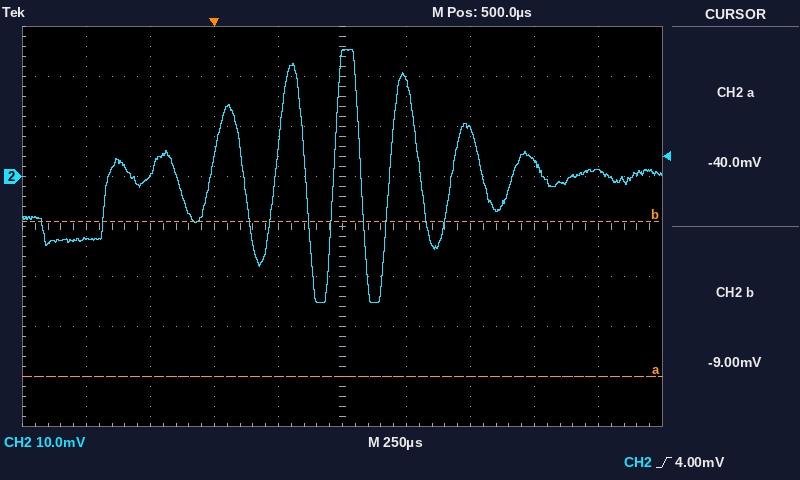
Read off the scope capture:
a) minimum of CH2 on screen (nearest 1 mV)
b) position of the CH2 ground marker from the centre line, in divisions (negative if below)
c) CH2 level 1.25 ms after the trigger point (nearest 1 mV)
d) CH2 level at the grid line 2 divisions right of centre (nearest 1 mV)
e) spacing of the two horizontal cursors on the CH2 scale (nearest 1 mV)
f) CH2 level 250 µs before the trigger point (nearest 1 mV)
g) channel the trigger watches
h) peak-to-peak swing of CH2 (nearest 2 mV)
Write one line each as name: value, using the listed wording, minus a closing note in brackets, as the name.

minimum of CH2 on screen: -25 mV
position of the CH2 ground marker from the centre line, in divisions: +1.0 div
CH2 level 1.25 ms after the trigger point: 3 mV
CH2 level at the grid line 2 divisions right of centre: 9 mV
spacing of the two horizontal cursors on the CH2 scale: 31 mV
CH2 level 250 µs before the trigger point: 0 mV
channel the trigger watches: CH2
peak-to-peak swing of CH2: 50 mV
